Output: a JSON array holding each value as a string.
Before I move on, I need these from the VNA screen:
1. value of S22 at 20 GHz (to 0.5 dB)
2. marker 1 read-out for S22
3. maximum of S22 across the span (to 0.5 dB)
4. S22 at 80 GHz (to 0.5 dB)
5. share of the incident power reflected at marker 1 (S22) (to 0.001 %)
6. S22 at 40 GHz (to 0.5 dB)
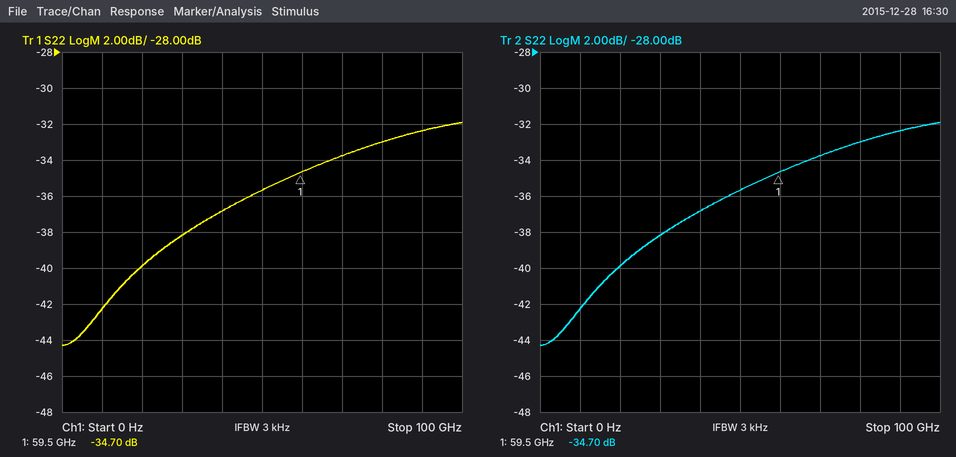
["-40.0 dB", "-34.70 dB", "-32.0 dB", "-33.0 dB", "0.034 %", "-37.0 dB"]
